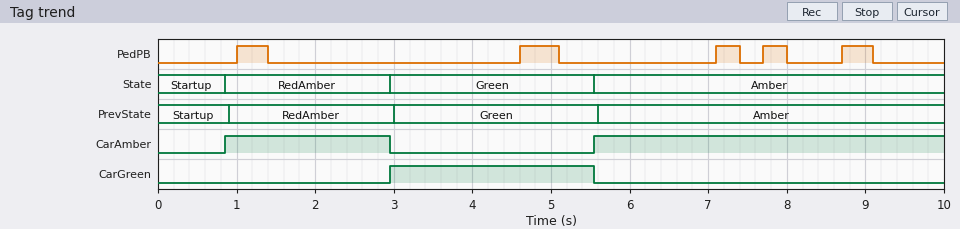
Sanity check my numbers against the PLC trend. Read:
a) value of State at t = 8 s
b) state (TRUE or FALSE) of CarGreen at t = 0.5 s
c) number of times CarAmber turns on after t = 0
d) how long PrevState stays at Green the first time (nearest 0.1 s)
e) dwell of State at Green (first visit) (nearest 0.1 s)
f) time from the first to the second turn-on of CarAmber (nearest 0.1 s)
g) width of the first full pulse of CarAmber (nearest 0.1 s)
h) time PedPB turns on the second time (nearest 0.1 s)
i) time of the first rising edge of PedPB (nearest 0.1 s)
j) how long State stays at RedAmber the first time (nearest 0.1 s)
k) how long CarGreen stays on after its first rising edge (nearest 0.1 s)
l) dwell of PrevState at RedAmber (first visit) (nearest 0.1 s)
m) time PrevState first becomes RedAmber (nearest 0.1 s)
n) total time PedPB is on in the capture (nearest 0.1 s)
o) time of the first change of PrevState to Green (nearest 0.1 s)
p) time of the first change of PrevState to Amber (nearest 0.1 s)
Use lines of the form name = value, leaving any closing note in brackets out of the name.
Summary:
value of State at t = 8 s = Amber
state (TRUE or FALSE) of CarGreen at t = 0.5 s = FALSE
number of times CarAmber turns on after t = 0 = 2
how long PrevState stays at Green the first time = 2.6 s
dwell of State at Green (first visit) = 2.6 s
time from the first to the second turn-on of CarAmber = 4.7 s
width of the first full pulse of CarAmber = 2.1 s
time PedPB turns on the second time = 4.6 s
time of the first rising edge of PedPB = 1.0 s
how long State stays at RedAmber the first time = 2.1 s
how long CarGreen stays on after its first rising edge = 2.6 s
dwell of PrevState at RedAmber (first visit) = 2.1 s
time PrevState first becomes RedAmber = 0.9 s
total time PedPB is on in the capture = 1.9 s
time of the first change of PrevState to Green = 3.0 s
time of the first change of PrevState to Amber = 5.6 s
